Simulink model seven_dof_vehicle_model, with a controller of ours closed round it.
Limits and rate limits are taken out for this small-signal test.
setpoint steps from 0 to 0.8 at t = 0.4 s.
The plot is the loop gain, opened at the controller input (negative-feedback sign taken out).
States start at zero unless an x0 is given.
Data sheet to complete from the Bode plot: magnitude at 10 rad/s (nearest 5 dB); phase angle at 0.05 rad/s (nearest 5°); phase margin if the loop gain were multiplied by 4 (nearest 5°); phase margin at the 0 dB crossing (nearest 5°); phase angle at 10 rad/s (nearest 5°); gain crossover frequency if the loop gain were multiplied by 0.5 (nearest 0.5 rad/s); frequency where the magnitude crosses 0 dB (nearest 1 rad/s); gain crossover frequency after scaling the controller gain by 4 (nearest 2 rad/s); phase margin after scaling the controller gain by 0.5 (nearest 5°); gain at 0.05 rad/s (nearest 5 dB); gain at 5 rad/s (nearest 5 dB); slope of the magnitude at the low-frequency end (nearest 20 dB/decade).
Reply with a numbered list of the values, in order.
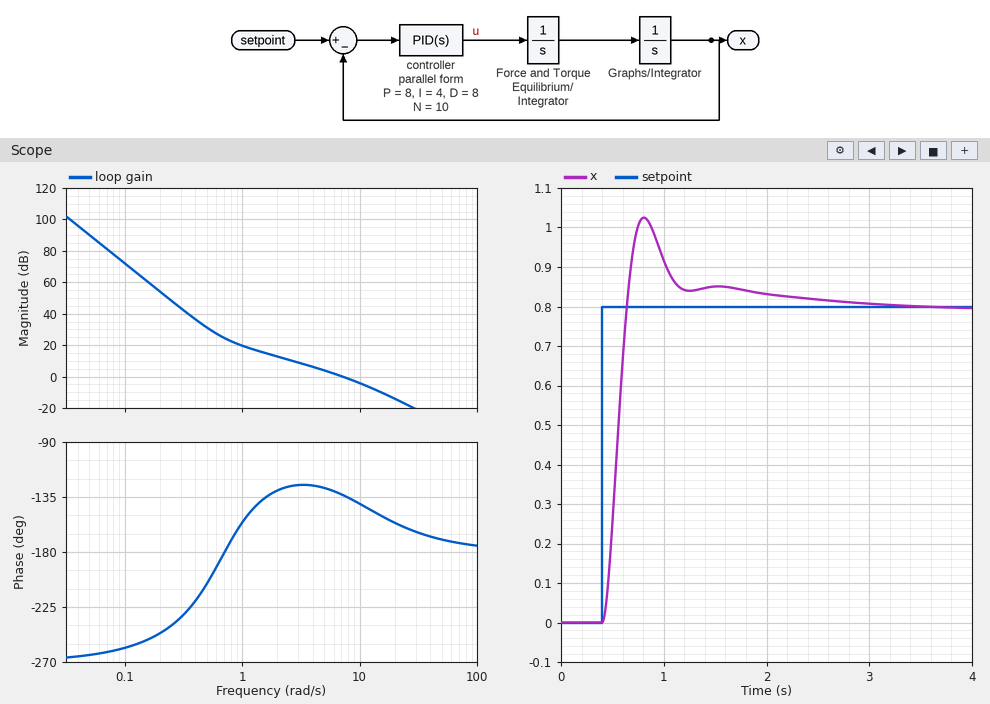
1. -5 dB
2. -265°
3. 25°
4. 45°
5. -140°
6. 4.0 rad/s
7. 7 rad/s
8. 18 rad/s
9. 55°
10. 90 dB
11. 5 dB
12. -60 dB/decade
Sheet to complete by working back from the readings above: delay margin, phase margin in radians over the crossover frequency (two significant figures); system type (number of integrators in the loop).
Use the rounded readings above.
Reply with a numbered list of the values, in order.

1. 0.11 s
2. 3
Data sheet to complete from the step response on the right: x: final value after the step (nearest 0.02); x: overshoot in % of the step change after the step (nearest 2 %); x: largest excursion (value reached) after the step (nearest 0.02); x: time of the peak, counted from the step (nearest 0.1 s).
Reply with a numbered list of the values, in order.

1. 0.80
2. 28 %
3. 1.02
4. 0.4 s
